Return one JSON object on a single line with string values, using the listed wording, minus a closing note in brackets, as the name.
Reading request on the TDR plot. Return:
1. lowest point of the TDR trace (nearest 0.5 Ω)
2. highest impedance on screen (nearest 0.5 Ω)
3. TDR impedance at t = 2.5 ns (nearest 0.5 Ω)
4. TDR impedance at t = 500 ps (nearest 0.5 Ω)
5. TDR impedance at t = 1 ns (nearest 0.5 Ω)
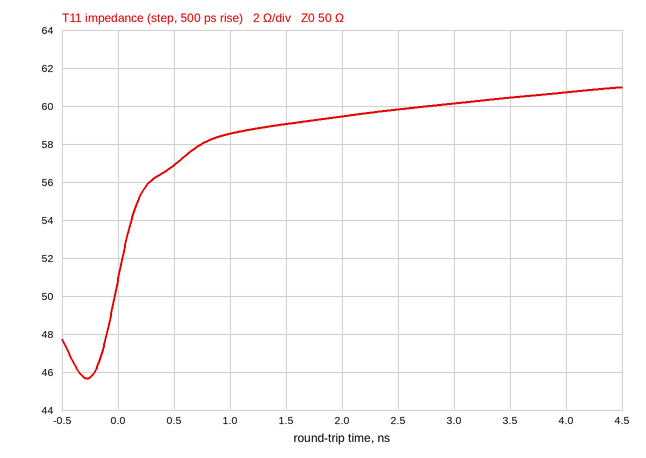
{"lowest point of the TDR trace": "45.5 Ω", "highest impedance on screen": "61.0 Ω", "TDR impedance at t = 2.5 ns": "60.0 Ω", "TDR impedance at t = 500 ps": "57.0 Ω", "TDR impedance at t = 1 ns": "58.5 Ω"}
